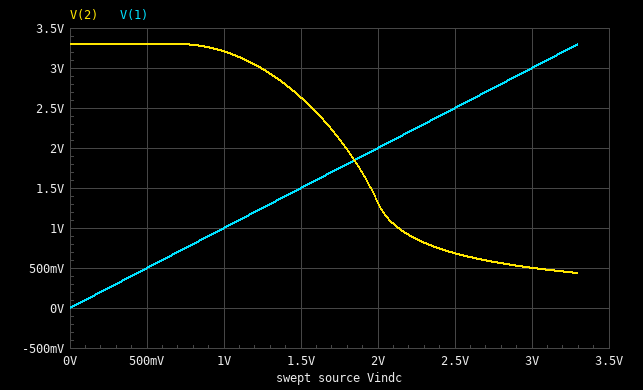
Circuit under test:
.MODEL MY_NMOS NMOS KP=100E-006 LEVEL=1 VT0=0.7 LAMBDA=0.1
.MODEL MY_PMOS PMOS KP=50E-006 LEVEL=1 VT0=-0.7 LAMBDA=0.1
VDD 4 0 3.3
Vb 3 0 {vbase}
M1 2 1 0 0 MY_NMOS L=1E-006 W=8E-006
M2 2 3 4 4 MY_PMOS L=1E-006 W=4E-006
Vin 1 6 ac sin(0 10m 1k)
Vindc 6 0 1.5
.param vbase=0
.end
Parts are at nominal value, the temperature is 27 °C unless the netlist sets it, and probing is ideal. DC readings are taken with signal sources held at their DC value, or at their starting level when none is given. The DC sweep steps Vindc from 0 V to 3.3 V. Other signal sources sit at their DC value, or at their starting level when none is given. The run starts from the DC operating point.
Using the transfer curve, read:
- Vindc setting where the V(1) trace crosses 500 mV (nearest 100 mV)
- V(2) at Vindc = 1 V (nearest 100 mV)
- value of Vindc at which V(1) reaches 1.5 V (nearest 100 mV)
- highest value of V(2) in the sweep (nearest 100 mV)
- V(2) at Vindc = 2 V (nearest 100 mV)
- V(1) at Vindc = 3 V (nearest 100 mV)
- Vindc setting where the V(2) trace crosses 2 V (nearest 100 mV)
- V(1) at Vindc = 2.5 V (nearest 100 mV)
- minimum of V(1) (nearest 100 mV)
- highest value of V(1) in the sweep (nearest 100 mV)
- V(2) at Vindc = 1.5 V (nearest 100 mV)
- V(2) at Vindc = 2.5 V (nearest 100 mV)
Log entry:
500 mV
3.2 V
1.5 V
3.3 V
1.3 V
3.0 V
1.8 V
2.5 V
0 V
3.3 V
2.6 V
700 mV
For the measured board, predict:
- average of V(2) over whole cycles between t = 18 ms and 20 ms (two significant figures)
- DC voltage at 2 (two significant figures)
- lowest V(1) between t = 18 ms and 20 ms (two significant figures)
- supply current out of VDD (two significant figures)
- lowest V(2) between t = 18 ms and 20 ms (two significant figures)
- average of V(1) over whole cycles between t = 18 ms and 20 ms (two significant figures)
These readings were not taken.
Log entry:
2.6 V
2.6 V
1.5 V
320 µA
2.6 V
1.5 V
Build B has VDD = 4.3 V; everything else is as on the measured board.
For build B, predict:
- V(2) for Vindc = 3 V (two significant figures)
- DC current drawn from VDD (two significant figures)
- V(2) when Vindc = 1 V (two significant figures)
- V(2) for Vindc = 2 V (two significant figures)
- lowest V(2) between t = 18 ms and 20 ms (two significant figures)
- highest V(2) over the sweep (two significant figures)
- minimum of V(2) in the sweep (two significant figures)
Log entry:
1.1 V
350 µA
4.2 V
3.0 V
3.8 V
4.3 V
920 mV
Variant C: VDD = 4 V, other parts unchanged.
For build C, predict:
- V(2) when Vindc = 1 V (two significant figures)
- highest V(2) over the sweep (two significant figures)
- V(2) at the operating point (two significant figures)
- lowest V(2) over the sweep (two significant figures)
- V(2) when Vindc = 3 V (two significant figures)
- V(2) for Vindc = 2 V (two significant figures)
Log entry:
3.9 V
4.0 V
3.5 V
750 mV
880 mV
2.6 V
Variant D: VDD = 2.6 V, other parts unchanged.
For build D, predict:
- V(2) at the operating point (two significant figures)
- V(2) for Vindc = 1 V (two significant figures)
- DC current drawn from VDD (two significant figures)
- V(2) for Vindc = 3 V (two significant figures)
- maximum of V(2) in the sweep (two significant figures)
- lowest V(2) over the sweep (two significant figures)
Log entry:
1.6 V
2.5 V
300 µA
250 mV
2.6 V
220 mV
